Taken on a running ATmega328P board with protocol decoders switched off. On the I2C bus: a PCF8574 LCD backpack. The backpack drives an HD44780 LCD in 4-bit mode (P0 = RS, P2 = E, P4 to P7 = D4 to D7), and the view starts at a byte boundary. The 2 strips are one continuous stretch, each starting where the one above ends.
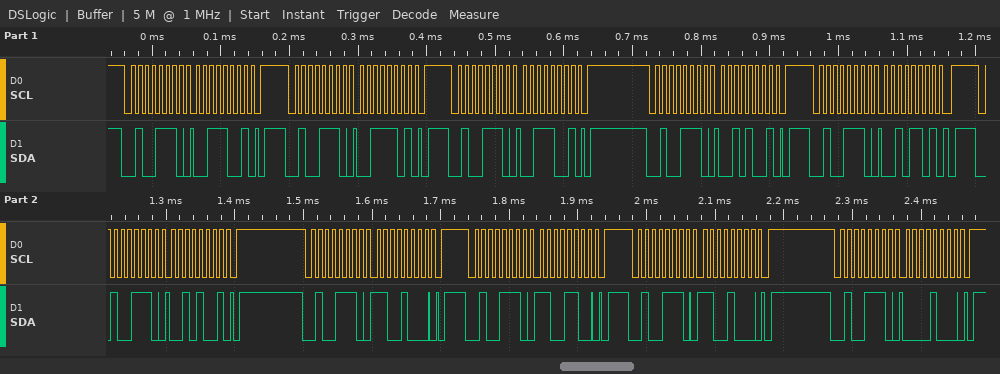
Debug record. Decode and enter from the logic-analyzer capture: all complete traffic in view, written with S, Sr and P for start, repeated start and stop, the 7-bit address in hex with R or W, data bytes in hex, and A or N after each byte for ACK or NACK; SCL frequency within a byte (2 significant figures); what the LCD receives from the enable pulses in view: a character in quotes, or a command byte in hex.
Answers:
S 27W A 39 A P S 27W A 3D A P S 27W A 39 A P S 27W A 29 A P S 27W A 2D A P S 27W A 29 A P S 27W A C8 A P S 27W A CC A P S 27W A C8 A P S 27W A 08 A P
100 kHz
'2'
